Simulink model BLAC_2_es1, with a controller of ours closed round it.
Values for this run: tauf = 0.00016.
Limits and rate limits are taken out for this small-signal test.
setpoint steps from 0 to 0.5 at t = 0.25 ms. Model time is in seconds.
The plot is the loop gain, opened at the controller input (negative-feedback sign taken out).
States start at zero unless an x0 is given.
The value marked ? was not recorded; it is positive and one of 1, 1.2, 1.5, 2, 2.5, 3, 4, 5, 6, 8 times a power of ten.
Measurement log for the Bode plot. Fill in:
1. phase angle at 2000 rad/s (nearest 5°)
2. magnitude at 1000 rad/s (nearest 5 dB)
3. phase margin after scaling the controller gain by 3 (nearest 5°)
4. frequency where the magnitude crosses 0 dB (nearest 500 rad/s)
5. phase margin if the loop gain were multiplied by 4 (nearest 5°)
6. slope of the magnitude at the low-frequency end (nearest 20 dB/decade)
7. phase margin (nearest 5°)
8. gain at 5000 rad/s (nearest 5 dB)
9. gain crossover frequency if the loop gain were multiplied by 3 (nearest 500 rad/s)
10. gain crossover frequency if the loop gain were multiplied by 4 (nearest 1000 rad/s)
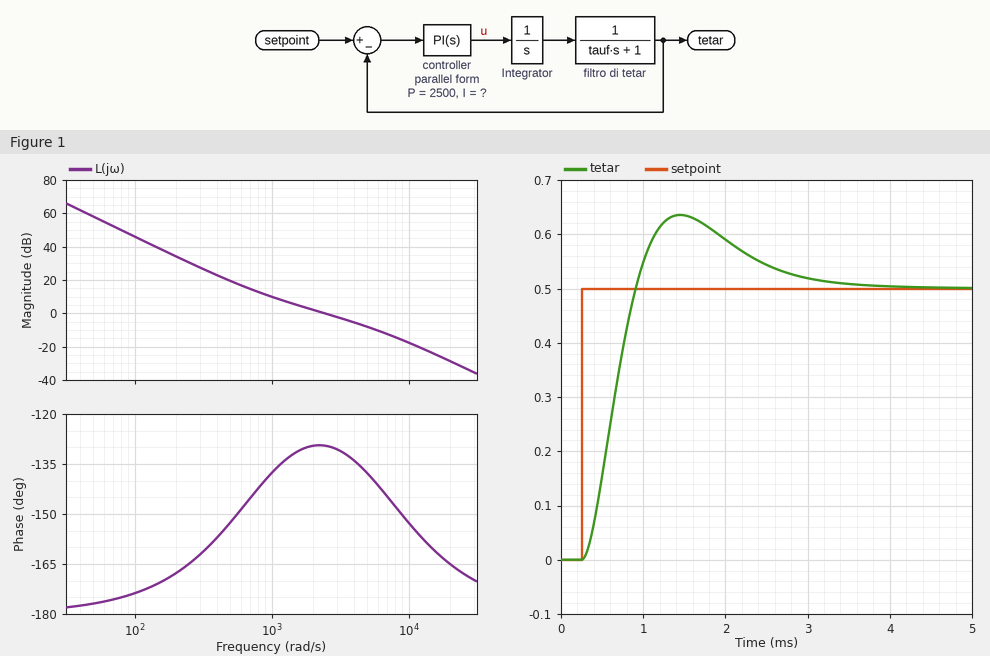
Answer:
-130°
10 dB
40°
2500 rad/s
35°
-40 dB/decade
50°
-10 dB
5500 rad/s
7000 rad/s
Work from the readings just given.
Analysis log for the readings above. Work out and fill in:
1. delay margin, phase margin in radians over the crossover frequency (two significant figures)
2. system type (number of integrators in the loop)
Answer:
0.00035 s
2
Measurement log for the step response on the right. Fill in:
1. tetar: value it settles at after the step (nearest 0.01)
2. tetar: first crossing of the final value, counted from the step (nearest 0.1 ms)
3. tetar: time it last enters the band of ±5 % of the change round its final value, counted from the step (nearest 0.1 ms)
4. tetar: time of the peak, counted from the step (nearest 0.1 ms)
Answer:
0.50
0.7 ms
2.6 ms
1.2 ms
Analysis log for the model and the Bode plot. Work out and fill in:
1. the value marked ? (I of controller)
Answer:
2e+06
